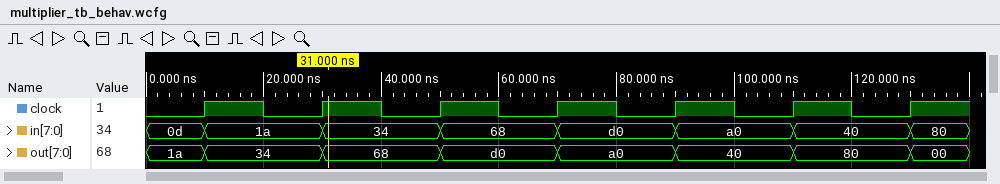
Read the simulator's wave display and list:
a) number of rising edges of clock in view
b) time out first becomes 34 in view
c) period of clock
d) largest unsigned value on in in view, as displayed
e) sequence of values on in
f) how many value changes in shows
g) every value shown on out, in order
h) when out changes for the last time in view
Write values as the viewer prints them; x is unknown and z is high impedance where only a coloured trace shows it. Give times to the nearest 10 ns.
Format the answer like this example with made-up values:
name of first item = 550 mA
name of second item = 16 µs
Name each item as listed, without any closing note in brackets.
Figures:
number of rising edges of clock in view = 7
time out first becomes 34 in view = 10 ns
period of clock = 20 ns
largest unsigned value on in in view, as displayed = d0
sequence of values on in = 0d, 1a, 34, 68, d0, a0, 40, 80
how many value changes in shows = 7
every value shown on out, in order = 1a, 34, 68, d0, a0, 40, 80, 00
when out changes for the last time in view = 130 ns
